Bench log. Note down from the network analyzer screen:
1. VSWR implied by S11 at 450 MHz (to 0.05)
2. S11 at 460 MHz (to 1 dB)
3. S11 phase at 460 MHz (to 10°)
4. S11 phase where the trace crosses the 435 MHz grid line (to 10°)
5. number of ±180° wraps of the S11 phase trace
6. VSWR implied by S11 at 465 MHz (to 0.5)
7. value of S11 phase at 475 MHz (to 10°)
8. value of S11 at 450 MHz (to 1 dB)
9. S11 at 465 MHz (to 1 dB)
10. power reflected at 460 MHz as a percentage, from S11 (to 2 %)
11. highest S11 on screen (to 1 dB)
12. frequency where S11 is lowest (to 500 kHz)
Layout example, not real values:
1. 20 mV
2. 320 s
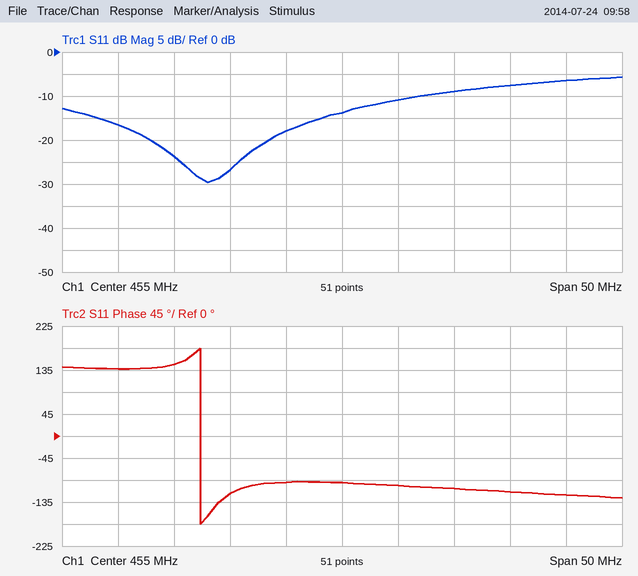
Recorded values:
1. 1.30
2. -11 dB
3. -100°
4. 140°
5. 1
6. 2.0
7. -120°
8. -18 dB
9. -9 dB
10. 8 %
11. -6 dB
12. 443.0 MHz
